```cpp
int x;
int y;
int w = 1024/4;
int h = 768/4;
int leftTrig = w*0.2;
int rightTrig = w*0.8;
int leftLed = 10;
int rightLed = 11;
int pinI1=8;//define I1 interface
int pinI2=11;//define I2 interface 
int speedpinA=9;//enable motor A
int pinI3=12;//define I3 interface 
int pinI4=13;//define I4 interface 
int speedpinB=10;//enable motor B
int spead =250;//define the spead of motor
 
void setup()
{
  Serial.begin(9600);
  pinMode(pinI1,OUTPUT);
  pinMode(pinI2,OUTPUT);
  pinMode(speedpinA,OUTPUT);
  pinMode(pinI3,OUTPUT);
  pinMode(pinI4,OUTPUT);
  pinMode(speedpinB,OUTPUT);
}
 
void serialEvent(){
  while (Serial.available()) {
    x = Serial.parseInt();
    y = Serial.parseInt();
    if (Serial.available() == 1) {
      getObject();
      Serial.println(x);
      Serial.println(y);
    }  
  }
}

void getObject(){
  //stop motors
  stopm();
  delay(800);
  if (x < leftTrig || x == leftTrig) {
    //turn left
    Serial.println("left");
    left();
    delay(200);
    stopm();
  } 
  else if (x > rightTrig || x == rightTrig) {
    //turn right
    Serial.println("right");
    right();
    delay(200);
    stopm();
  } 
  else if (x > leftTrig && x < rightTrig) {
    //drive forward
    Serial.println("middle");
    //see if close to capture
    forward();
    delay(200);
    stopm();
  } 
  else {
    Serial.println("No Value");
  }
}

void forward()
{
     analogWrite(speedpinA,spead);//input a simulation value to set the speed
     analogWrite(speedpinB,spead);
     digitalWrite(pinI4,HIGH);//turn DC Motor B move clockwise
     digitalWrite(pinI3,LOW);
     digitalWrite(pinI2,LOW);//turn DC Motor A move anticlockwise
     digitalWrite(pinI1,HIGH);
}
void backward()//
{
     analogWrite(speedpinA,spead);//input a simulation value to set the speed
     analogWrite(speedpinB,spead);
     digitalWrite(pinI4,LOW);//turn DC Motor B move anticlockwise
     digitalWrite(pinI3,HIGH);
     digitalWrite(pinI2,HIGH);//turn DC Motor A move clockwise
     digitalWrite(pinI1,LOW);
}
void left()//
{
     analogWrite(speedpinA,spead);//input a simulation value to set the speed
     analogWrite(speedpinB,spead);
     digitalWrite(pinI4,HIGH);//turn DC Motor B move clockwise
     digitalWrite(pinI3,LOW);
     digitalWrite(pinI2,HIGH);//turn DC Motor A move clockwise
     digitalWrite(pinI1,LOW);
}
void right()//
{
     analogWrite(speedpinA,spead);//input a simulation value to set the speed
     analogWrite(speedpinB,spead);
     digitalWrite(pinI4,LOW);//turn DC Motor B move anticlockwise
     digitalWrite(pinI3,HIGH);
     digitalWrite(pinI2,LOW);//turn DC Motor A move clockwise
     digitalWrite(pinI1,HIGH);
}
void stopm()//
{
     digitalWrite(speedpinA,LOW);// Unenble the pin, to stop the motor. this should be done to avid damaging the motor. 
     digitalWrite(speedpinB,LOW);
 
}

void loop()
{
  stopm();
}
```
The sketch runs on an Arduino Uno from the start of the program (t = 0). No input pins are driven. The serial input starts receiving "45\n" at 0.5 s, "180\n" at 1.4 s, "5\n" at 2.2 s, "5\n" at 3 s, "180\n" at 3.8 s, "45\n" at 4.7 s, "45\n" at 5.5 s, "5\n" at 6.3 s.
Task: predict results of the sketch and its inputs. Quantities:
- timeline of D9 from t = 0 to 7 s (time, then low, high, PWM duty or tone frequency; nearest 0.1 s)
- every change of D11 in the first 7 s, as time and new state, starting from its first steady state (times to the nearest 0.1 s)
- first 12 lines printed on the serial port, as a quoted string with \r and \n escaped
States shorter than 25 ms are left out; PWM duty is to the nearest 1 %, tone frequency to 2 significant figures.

0 s low; 2.2 s PWM 98 %; 2.4 s low; 3.8 s PWM 98 %; 4 s low; 5.5 s PWM 98 %; 5.7 s low
0 s low; 2.2 s high; 5.5 s low
"left\r\n45\r\n180\r\nleft\r\n5\r\n5\r\nmiddle\r\n180\r\n45\r\nleft\r\n45\r\n5\r\n"
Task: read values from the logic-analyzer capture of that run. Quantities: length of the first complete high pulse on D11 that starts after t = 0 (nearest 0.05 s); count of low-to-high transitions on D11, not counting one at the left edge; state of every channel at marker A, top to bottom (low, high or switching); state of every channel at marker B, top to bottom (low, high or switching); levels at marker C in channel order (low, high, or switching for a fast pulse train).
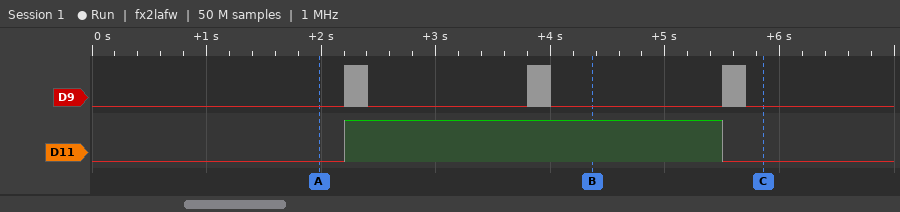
3.30 s
1
D9 low, D11 low
D9 low, D11 high
D9 low, D11 low
